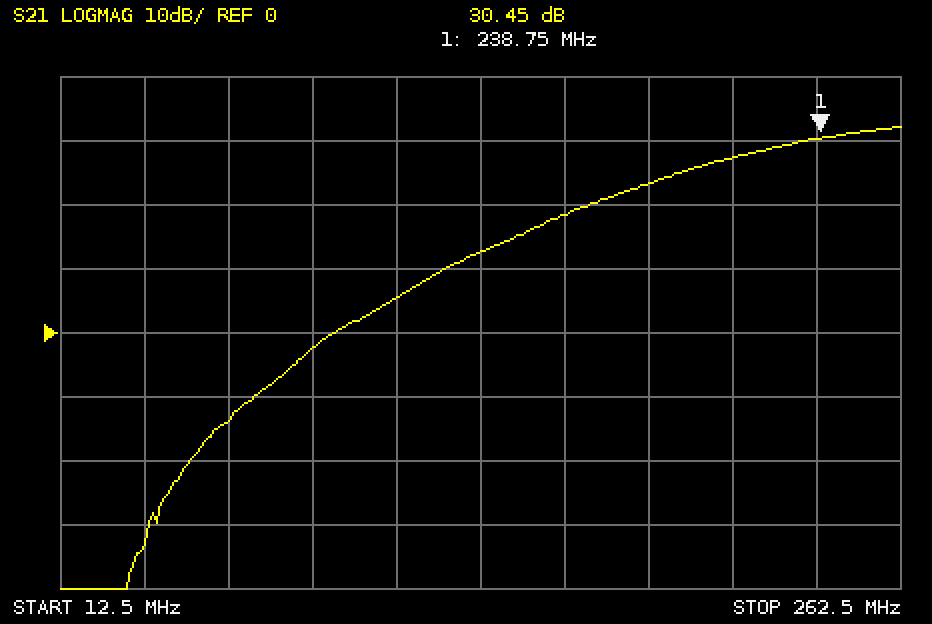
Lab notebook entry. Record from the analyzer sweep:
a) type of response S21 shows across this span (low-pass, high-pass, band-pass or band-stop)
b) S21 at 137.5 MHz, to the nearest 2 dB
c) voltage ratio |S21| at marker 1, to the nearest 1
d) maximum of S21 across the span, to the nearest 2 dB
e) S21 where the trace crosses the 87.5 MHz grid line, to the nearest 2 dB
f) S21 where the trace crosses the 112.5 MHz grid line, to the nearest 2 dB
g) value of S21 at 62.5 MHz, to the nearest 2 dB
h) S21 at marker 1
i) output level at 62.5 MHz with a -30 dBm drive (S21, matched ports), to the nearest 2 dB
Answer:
high-pass
12 dB
33
32 dB
-2 dB
6 dB
-14 dB
30.45 dB
-44 dBm
